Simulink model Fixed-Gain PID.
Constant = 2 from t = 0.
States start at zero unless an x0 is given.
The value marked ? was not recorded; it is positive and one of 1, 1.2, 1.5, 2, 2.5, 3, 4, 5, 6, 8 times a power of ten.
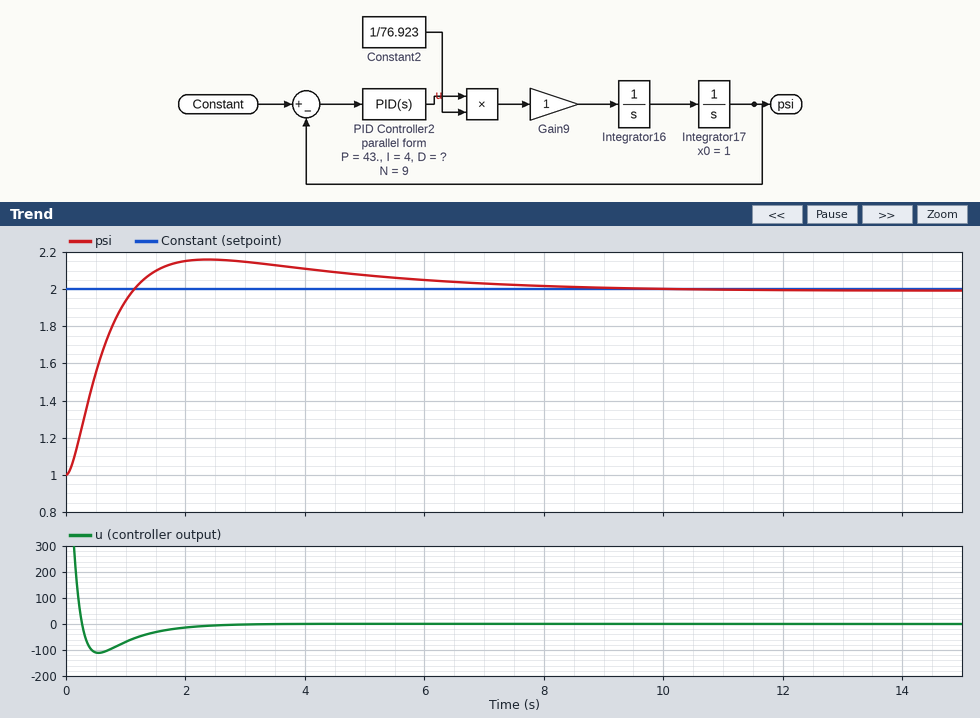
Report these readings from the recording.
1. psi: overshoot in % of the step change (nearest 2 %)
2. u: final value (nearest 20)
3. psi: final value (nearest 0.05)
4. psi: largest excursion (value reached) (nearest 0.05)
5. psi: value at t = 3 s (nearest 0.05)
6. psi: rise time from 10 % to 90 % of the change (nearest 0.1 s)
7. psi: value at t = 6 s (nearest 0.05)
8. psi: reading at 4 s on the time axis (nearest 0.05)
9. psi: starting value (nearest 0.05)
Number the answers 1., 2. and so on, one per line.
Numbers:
1. 16 %
2. 0
3. 2.00
4. 2.15
5. 2.15
6. 0.8 s
7. 2.05
8. 2.10
9. 1.00
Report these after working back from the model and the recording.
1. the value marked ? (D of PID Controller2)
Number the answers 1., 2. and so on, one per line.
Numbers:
1. 120
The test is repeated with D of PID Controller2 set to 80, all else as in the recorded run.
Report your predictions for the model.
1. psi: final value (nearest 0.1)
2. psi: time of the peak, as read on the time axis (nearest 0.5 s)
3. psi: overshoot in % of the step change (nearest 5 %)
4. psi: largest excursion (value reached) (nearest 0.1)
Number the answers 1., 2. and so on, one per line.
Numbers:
1. 2.0
2. 3.0 s
3. 25 %
4. 2.3
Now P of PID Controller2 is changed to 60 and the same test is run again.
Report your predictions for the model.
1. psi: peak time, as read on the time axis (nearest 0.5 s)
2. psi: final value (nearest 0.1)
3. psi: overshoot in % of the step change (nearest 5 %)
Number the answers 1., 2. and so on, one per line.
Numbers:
1. 2.0 s
2. 2.0
3. 20 %
